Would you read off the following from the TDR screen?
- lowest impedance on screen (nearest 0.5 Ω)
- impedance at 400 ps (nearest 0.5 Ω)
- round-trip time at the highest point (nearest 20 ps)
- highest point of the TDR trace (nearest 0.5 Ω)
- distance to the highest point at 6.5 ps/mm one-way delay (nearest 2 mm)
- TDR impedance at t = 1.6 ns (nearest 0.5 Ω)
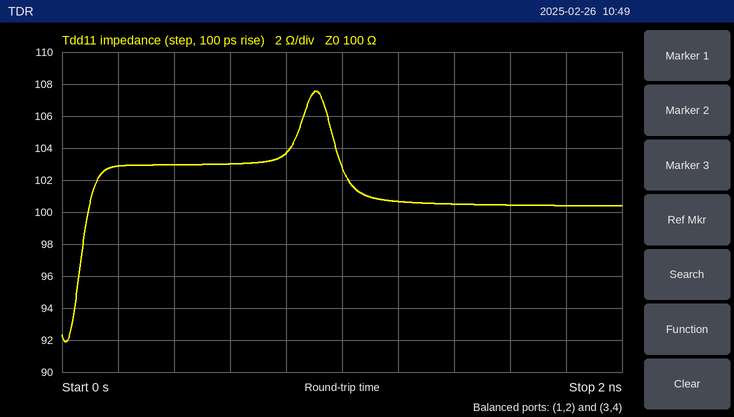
92.0 Ω
103.0 Ω
900 ps
107.5 Ω
70 mm
100.5 Ω
